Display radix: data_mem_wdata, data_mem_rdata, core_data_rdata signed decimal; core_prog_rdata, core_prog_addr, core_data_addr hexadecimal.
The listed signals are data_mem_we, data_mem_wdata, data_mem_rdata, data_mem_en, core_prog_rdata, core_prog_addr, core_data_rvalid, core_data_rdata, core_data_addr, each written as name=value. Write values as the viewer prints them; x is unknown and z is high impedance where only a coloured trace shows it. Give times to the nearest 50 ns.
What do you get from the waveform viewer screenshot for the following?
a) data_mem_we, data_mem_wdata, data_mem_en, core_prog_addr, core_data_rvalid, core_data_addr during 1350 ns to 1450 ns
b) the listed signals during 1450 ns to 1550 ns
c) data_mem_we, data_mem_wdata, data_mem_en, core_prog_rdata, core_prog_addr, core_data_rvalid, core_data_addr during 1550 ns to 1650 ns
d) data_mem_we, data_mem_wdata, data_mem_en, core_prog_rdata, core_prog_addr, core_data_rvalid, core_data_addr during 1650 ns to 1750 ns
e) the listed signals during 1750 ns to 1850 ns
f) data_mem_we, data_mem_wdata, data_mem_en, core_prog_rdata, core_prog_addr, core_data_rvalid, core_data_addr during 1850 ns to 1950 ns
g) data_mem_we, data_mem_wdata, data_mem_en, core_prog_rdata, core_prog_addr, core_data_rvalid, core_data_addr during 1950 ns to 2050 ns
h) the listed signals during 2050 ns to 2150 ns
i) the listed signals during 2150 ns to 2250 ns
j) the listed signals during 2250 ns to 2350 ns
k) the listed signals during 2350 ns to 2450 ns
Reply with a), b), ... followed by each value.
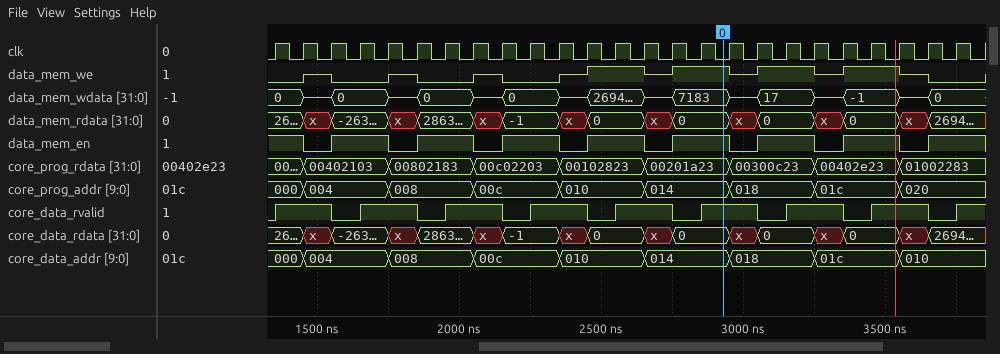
a) data_mem_we=0, data_mem_wdata=0, data_mem_en=1, core_prog_addr=000, core_data_rvalid=1, core_data_addr=000
b) data_mem_we=z, data_mem_wdata=z, data_mem_rdata=x, data_mem_en=0, core_prog_rdata=00402103, core_prog_addr=004, core_data_rvalid=1, core_data_rdata=x, core_data_addr=004
c) data_mem_we=0, data_mem_wdata=0, data_mem_en=1, core_prog_rdata=00402103, core_prog_addr=004, core_data_rvalid=0, core_data_addr=004
d) data_mem_we=0, data_mem_wdata=0, data_mem_en=1, core_prog_rdata=00402103, core_prog_addr=004, core_data_rvalid=1, core_data_addr=004
e) data_mem_we=z, data_mem_wdata=z, data_mem_rdata=x, data_mem_en=0, core_prog_rdata=00802183, core_prog_addr=008, core_data_rvalid=1, core_data_rdata=x, core_data_addr=008
f) data_mem_we=0, data_mem_wdata=0, data_mem_en=1, core_prog_rdata=00802183, core_prog_addr=008, core_data_rvalid=0, core_data_addr=008
g) data_mem_we=0, data_mem_wdata=0, data_mem_en=1, core_prog_rdata=00802183, core_prog_addr=008, core_data_rvalid=1, core_data_addr=008
h) data_mem_we=z, data_mem_wdata=z, data_mem_rdata=x, data_mem_en=0, core_prog_rdata=00c02203, core_prog_addr=00c, core_data_rvalid=1, core_data_rdata=x, core_data_addr=00c
i) data_mem_we=0, data_mem_wdata=0, data_mem_rdata=-1, data_mem_en=1, core_prog_rdata=00c02203, core_prog_addr=00c, core_data_rvalid=0, core_data_rdata=-1, core_data_addr=00c
j) data_mem_we=0, data_mem_wdata=0, data_mem_rdata=-1, data_mem_en=1, core_prog_rdata=00c02203, core_prog_addr=00c, core_data_rvalid=1, core_data_rdata=-1, core_data_addr=00c
k) data_mem_we=z, data_mem_wdata=z, data_mem_rdata=x, data_mem_en=0, core_prog_rdata=00102823, core_prog_addr=010, core_data_rvalid=1, core_data_rdata=x, core_data_addr=010
